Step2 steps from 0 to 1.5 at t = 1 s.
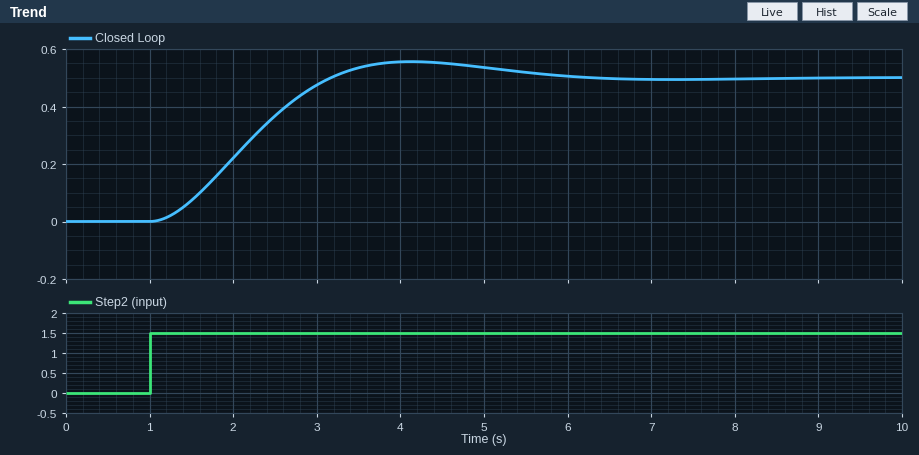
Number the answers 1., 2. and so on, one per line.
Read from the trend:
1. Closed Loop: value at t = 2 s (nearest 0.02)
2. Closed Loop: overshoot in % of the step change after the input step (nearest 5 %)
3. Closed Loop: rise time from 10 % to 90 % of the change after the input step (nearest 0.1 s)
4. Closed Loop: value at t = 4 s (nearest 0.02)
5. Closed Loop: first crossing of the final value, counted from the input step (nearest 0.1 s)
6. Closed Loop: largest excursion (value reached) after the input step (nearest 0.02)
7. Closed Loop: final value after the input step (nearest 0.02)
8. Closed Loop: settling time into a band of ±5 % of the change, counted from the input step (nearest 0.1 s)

1. 0.22
2. 10 %
3. 1.5 s
4. 0.56
5. 2.2 s
6. 0.56
7. 0.50
8. 4.3 s
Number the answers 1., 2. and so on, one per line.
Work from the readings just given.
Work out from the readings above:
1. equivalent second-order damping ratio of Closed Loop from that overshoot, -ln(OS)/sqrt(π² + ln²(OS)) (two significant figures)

1. 0.59
